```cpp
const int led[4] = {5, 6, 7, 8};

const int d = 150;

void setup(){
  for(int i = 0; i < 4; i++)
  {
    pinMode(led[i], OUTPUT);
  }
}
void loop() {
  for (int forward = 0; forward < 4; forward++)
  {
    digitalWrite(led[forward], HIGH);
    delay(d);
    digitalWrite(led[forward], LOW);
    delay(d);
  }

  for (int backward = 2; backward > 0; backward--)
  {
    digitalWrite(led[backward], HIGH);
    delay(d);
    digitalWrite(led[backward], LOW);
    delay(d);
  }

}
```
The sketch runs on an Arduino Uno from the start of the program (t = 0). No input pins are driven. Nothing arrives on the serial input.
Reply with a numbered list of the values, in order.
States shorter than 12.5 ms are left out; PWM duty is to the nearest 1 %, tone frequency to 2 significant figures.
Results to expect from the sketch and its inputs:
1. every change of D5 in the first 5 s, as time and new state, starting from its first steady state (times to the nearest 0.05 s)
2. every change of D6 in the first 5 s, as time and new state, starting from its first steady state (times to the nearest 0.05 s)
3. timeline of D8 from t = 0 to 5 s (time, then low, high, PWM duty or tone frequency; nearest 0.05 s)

1. 0 s high; 0.15 s low; 1.8 s high; 1.95 s low; 3.6 s high; 3.75 s low
2. 0 s low; 0.3 s high; 0.45 s low; 1.5 s high; 1.65 s low; 2.1 s high; 2.25 s low; 3.3 s high; 3.45 s low; 3.9 s high; 4.05 s low
3. 0 s low; 0.9 s high; 1.05 s low; 2.7 s high; 2.85 s low; 4.5 s high; 4.65 s low
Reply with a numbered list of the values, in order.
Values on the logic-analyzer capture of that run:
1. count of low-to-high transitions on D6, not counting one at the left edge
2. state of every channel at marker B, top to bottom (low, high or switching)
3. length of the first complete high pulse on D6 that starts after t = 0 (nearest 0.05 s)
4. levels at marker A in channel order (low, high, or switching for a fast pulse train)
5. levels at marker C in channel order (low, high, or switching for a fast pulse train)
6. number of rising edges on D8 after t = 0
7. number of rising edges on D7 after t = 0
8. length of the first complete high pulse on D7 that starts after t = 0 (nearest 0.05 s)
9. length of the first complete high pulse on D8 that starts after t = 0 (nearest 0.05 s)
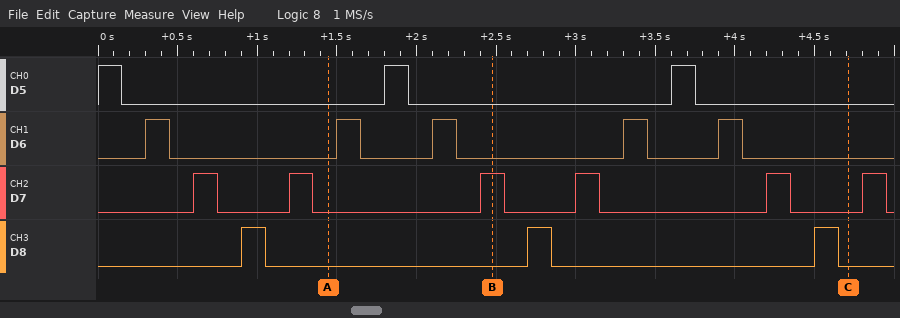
1. 5
2. D5 low, D6 low, D7 high, D8 low
3. 0.15 s
4. D5 low, D6 low, D7 low, D8 low
5. D5 low, D6 low, D7 low, D8 low
6. 3
7. 6
8. 0.15 s
9. 0.15 s
